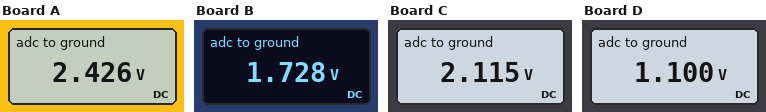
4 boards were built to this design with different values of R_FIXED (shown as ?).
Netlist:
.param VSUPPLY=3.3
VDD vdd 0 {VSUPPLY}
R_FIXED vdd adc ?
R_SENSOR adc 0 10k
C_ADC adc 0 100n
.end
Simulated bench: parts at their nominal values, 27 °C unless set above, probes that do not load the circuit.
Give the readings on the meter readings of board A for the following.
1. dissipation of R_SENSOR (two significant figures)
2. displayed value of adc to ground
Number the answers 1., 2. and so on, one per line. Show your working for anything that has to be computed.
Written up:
1. (2.426 V)^2 / 10 kΩ = 590 µW
2. 2.426 V
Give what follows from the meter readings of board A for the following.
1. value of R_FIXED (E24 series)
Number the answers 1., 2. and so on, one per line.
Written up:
1. 3.6 kΩ
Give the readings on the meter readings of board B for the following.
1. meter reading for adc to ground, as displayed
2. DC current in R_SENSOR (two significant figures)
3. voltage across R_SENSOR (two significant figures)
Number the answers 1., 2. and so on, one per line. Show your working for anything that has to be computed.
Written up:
1. 1.728 V
2. (1.728 V) / 10 kΩ = 170 µA
3. 1.728 V = 1.7 V
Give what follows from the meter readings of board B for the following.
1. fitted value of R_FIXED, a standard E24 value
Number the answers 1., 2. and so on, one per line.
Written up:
1. 9.1 kΩ
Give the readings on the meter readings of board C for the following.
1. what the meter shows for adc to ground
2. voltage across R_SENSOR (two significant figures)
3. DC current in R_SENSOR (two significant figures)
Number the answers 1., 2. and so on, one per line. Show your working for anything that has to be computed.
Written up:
1. 2.115 V
2. 2.115 V = 2.1 V
3. (2.115 V) / 10 kΩ = 210 µA
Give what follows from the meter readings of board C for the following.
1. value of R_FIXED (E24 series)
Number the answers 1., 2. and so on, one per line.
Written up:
1. 5.6 kΩ
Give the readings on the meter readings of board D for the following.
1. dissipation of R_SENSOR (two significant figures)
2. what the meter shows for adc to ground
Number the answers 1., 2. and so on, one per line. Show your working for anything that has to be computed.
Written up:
1. (1.1 V)^2 / 10 kΩ = 120 µW
2. 1.100 V
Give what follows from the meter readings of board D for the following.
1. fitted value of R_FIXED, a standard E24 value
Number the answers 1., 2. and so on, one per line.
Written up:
1. 20 kΩ
